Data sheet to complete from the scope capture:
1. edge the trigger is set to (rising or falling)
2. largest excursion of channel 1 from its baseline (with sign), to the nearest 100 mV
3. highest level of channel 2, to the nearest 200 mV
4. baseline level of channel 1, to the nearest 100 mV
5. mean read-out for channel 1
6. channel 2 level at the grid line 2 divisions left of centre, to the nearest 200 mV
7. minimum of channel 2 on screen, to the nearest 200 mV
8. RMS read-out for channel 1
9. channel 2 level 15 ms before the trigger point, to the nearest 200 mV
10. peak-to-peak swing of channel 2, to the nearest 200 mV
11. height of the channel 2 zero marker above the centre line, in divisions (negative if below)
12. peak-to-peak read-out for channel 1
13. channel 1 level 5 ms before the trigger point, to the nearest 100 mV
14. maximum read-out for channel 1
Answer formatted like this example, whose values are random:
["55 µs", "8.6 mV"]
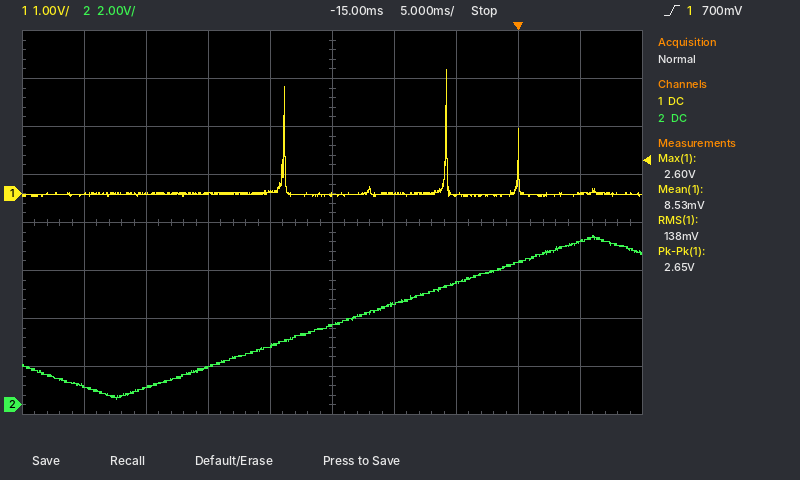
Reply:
["rising", "+2.6 V", "7.0 V", "0.0 V", "8.53 mV", "1.6 V", "200 mV", "138 mV", "3.4 V", "6.8 V", "-3.8 div", "2.65 V", "0.0 V", "2.60 V"]
